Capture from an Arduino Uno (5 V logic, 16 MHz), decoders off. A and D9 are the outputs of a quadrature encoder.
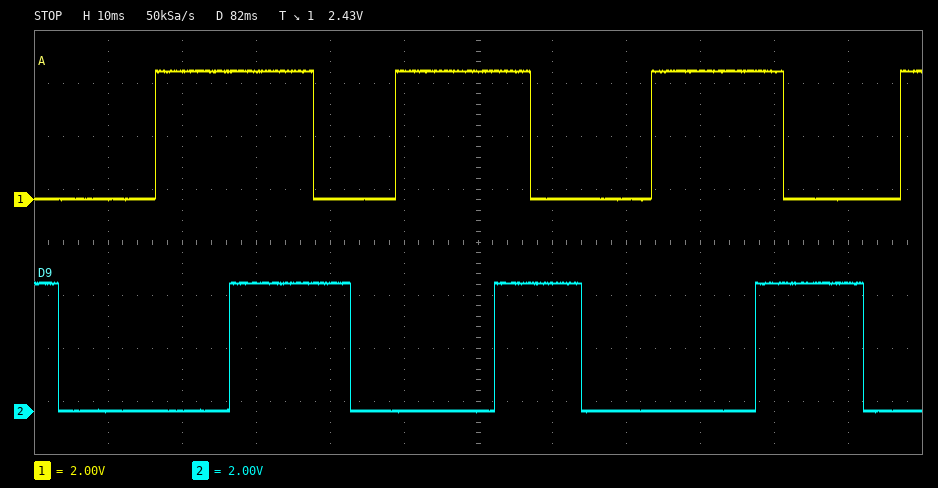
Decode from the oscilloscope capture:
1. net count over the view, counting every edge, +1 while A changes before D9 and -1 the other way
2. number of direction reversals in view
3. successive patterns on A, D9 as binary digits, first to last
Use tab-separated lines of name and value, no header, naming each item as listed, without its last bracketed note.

net count over the view, counting every edge, +1 while A changes before D9 and -1 the other way	+14
number of direction reversals in view	0
successive patterns on A, D9 as binary digits, first to last	01 00 10 11 01 00 10 11 01 00 10 11 01 00 10
